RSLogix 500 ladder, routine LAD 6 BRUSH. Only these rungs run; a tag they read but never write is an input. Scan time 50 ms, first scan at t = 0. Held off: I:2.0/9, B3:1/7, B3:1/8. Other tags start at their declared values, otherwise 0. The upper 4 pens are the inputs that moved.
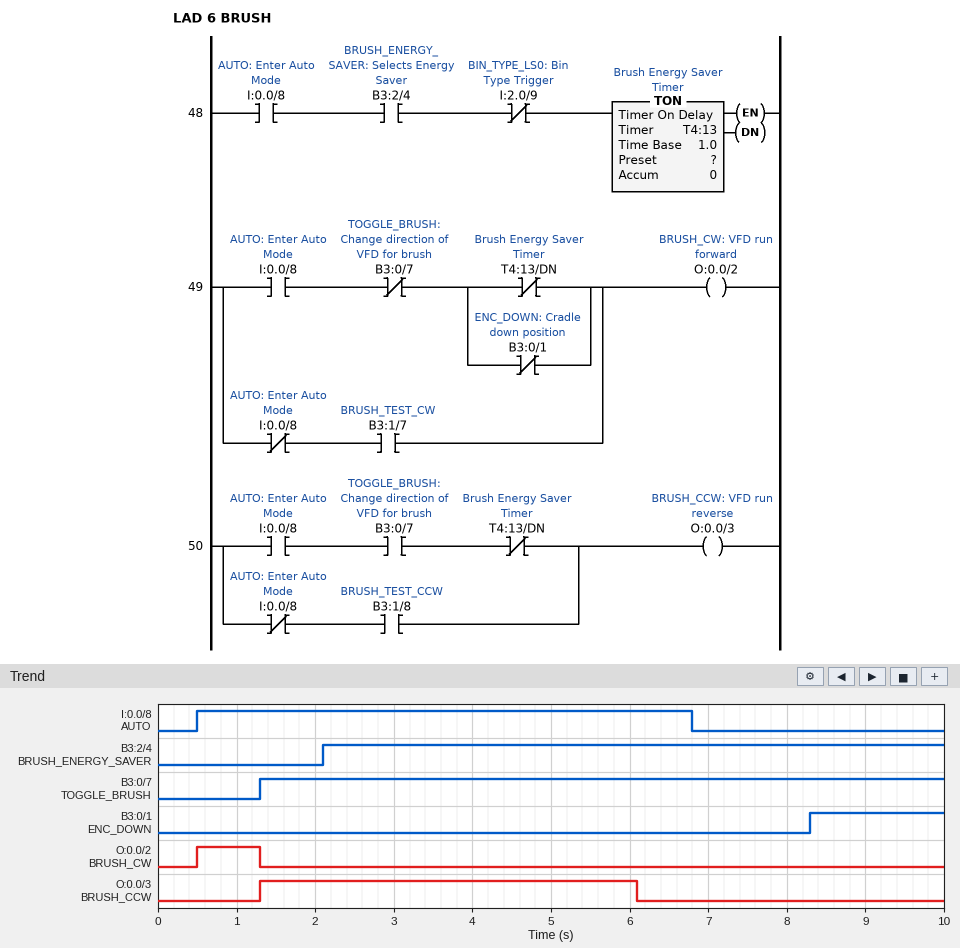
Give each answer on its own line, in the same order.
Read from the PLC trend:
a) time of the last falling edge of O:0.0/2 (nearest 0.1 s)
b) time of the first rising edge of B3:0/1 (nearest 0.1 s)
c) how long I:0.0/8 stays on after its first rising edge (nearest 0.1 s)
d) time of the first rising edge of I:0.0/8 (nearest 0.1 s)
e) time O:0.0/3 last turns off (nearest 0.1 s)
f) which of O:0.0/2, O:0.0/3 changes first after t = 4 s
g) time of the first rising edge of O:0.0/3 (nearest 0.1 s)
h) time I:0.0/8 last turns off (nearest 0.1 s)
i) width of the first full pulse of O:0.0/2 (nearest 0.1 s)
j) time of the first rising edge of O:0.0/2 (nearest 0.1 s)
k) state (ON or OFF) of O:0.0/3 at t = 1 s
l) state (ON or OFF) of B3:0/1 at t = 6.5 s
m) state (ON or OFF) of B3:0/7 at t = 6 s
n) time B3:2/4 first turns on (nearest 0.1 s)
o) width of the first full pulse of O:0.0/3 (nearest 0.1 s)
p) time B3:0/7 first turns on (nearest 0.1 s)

1.3 s
8.3 s
6.3 s
0.5 s
6.1 s
O:0.0/3
1.3 s
6.8 s
0.8 s
0.5 s
OFF
OFF
ON
2.1 s
4.8 s
1.3 s
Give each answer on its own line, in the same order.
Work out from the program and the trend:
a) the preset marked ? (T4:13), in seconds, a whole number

4 s
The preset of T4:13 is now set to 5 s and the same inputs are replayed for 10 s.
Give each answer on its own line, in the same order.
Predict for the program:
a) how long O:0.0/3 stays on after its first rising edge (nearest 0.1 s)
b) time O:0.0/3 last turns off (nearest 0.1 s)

5.5 s
6.8 s
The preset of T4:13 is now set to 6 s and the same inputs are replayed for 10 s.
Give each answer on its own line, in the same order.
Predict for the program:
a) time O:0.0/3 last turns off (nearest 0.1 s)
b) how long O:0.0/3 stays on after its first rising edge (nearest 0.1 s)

6.8 s
5.5 s
